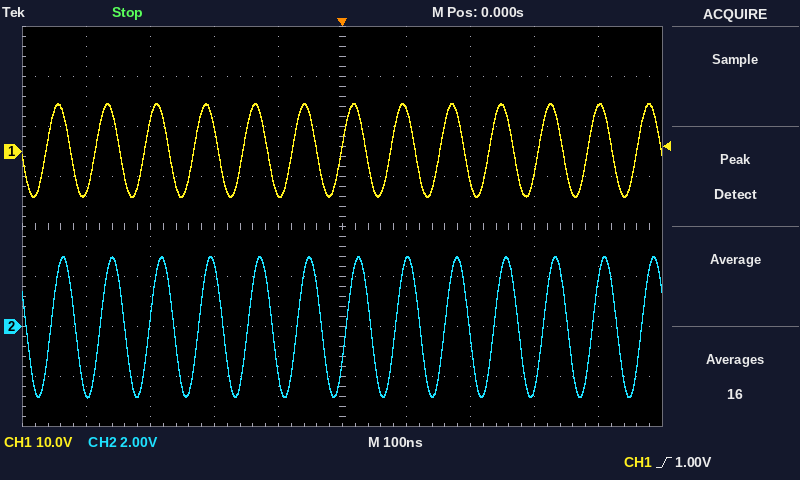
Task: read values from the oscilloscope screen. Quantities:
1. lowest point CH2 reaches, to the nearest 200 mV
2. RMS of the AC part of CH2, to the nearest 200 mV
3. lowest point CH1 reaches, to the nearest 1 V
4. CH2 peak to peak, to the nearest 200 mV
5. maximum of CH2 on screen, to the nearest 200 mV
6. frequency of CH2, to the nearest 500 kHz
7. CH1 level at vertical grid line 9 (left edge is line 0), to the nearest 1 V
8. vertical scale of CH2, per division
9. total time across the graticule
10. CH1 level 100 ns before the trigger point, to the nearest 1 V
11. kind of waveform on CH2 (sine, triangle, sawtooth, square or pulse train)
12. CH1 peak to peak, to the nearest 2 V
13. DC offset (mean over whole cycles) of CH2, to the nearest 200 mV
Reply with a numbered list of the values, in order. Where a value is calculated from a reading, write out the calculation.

1. -2.8 V
2. 5.6 V / (2√2) ≈ 2.0 V
3. -9 V
4. 2.8 V − (-2.8 V) = 5.6 V
5. 2.8 V
6. 13.0 MHz
7. 9 V
8. 2 V
9. 1 µs
10. -8 V
11. sine
12. 18 V
13. (2.8 V + (-2.8 V)) / 2 ≈ 0.0 V
